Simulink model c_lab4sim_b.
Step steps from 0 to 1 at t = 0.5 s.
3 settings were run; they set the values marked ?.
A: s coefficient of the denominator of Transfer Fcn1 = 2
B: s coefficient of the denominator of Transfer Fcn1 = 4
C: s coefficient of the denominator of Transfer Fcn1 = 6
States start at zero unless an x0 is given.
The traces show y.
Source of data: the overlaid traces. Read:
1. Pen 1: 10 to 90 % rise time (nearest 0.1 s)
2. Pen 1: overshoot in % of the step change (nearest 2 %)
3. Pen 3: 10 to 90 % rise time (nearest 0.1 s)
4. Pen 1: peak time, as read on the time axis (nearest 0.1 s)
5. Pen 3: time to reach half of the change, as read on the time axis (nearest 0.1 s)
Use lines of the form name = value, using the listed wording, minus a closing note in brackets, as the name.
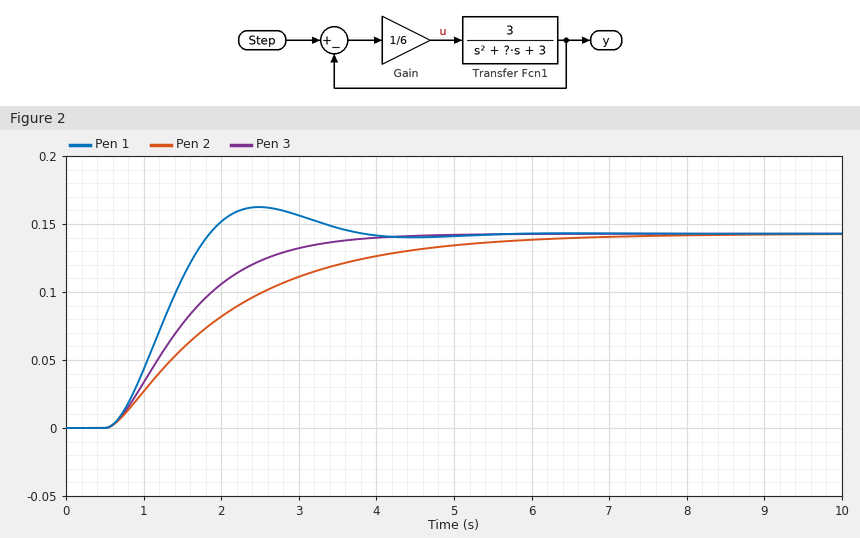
Pen 1: 10 to 90 % rise time = 0.9 s
Pen 1: overshoot in % of the step change = 14 %
Pen 3: 10 to 90 % rise time = 2.0 s
Pen 1: peak time, as read on the time axis = 2.5 s
Pen 3: time to reach half of the change, as read on the time axis = 1.4 s
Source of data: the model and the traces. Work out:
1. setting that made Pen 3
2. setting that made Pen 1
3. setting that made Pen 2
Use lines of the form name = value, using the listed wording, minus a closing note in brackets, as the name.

setting that made Pen 3 = B
setting that made Pen 1 = A
setting that made Pen 2 = C
